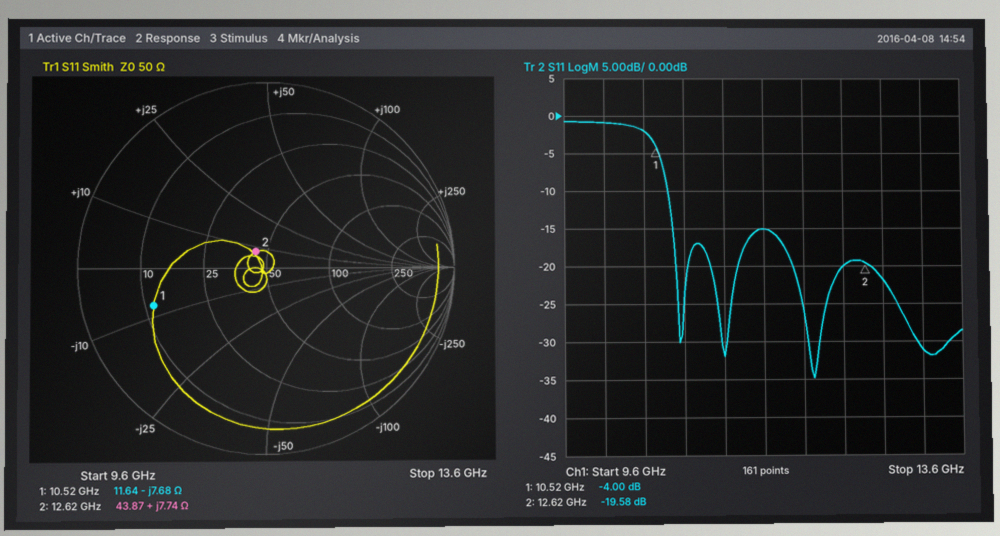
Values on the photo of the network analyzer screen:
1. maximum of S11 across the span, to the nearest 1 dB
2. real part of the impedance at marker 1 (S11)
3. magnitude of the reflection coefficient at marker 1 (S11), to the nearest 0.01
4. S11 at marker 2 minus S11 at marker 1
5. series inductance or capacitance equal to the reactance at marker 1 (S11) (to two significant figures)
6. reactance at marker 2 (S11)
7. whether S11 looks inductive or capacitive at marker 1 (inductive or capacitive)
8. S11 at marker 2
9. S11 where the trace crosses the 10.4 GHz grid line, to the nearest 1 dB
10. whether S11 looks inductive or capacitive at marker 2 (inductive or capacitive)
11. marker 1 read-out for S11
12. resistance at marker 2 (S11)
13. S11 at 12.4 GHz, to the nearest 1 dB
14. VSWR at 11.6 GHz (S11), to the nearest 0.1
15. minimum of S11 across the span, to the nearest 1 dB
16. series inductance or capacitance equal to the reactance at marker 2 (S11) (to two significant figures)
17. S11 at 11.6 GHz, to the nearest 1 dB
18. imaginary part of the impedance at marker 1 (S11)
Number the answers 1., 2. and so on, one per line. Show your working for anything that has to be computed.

1. -1 dB
2. 11.64 Ω
3. 0.63
4. -19.58 − (-4) = -15.58 dB
5. C = 1/(2π × 10.52 GHz × 7.68 Ω) ≈ 2.0 pF
6. +7.74 Ω
7. capacitive
8. -19.58 dB
9. -2 dB
10. inductive
11. -4.00 dB
12. 43.87 Ω
13. -20 dB
14. |Γ| = 10^(-15/20) = 0.1778; VSWR = (1 + 0.1778)/(1 − 0.1778) ≈ 1.4
15. -35 dB
16. L = 7.74 Ω/(2π × 12.62 GHz) ≈ 98 pH
17. -15 dB
18. -7.68 Ω
